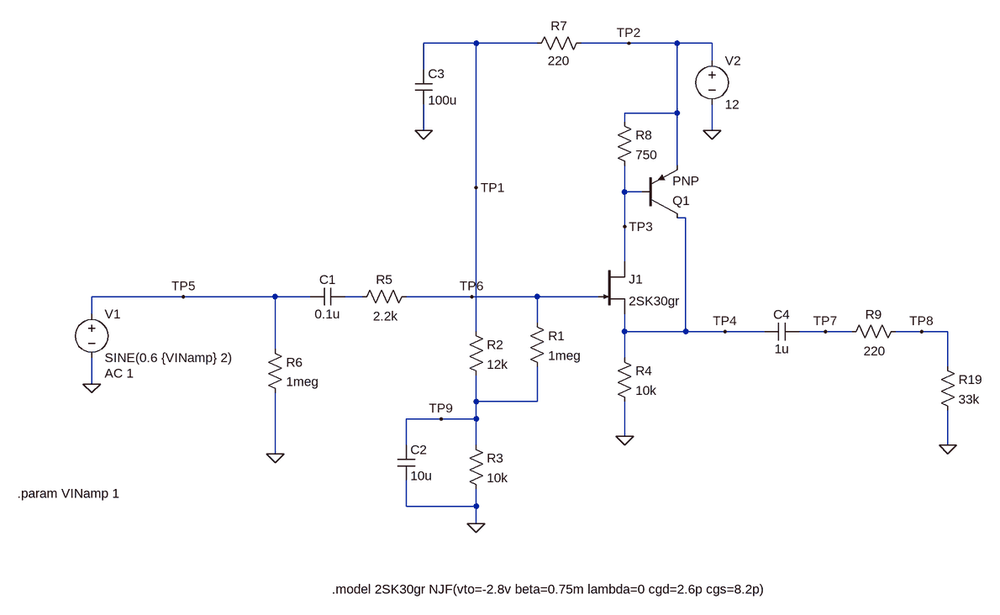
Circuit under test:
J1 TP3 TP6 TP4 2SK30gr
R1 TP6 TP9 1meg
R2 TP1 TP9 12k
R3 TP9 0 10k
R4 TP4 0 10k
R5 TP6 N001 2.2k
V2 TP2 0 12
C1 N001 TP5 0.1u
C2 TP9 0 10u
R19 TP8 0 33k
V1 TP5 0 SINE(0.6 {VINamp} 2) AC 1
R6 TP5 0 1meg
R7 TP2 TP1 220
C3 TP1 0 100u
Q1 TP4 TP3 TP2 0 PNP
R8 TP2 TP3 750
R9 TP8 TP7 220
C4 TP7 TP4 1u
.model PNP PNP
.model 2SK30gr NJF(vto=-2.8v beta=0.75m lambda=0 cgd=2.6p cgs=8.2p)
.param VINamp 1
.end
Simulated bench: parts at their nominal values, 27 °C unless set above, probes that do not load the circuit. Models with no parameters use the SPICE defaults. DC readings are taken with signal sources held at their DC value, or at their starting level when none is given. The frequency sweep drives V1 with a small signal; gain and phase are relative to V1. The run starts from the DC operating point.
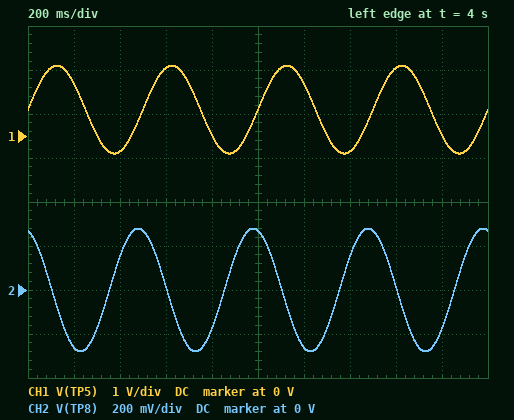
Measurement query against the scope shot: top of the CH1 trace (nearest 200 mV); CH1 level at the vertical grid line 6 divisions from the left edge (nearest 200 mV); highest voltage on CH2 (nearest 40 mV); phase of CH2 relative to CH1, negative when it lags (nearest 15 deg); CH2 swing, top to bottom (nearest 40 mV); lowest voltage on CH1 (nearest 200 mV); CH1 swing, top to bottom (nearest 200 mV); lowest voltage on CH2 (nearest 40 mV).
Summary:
1.6 V
1.2 V
280 mV
105 deg
560 mV
-400 mV
2.0 V
-280 mV
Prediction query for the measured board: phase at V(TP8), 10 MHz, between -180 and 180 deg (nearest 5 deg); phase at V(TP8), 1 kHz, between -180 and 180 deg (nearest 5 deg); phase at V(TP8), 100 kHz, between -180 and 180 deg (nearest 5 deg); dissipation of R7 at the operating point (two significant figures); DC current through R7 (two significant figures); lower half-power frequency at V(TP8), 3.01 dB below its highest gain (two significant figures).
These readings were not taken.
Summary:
-10 deg
0 deg
0 deg
64 µW
540 µA
5.2 Hz
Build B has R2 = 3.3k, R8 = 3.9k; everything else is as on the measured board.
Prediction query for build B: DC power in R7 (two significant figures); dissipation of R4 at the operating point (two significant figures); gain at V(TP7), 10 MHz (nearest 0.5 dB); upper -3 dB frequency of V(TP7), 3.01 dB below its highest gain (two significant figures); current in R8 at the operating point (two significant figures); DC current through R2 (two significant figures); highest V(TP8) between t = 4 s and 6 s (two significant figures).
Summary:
170 µW
12 mW
-10.0 dB
21 MHz
200 µA
890 µA
200 mV
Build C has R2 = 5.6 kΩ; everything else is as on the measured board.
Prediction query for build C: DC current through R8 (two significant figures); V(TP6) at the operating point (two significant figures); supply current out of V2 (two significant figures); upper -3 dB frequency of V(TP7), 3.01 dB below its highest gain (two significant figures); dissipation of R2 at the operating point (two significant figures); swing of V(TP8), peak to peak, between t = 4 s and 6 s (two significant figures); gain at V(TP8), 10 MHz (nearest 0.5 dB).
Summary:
900 µA
7.6 V
1.7 mA
41 MHz
3.2 mW
580 mV
-0.5 dB
